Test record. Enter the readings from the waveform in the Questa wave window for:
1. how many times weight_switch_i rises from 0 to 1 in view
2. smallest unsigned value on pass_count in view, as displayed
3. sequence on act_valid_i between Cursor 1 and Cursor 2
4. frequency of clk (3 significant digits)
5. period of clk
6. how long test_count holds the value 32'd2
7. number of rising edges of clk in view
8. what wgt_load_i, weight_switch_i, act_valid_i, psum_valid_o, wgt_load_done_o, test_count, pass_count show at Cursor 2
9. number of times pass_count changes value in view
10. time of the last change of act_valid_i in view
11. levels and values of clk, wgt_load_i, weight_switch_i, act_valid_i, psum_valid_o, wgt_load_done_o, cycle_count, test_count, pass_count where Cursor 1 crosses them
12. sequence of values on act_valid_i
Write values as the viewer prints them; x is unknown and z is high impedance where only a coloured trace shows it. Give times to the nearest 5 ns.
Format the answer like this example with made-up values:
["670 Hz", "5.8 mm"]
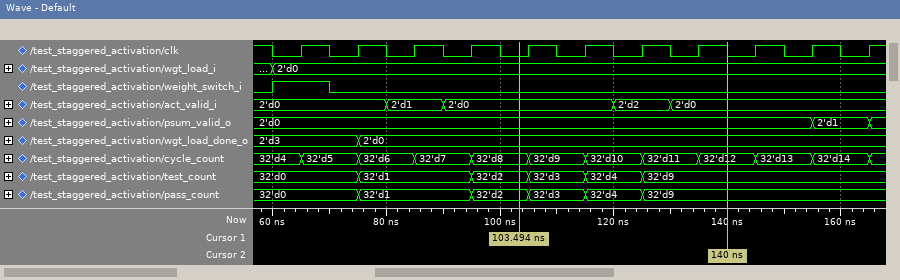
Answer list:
["1", "32'd0", "2'd0, 2'd2, 2'd0", "100 MHz", "10 ns", "10 ns", "11", "wgt_load_i=2'd0, weight_switch_i=0, act_valid_i=2'd0, psum_valid_o=2'd0, wgt_load_done_o=2'd0, test_count=32'd9, pass_count=32'd9", "5", "130 ns", "clk=0, wgt_load_i=2'd0, weight_switch_i=0, act_valid_i=2'd0, psum_valid_o=2'd0, wgt_load_done_o=2'd0, cycle_count=32'd8, test_count=32'd2, pass_count=32'd2", "2'd0, 2'd1, 2'd0, 2'd2, 2'd0"]
